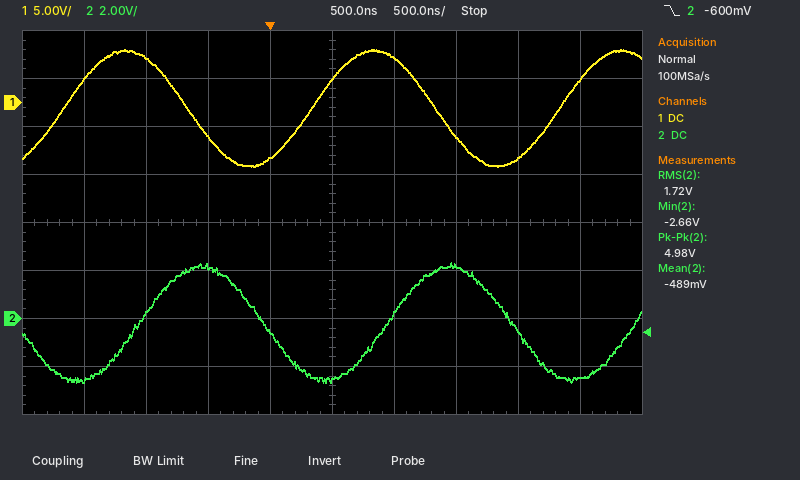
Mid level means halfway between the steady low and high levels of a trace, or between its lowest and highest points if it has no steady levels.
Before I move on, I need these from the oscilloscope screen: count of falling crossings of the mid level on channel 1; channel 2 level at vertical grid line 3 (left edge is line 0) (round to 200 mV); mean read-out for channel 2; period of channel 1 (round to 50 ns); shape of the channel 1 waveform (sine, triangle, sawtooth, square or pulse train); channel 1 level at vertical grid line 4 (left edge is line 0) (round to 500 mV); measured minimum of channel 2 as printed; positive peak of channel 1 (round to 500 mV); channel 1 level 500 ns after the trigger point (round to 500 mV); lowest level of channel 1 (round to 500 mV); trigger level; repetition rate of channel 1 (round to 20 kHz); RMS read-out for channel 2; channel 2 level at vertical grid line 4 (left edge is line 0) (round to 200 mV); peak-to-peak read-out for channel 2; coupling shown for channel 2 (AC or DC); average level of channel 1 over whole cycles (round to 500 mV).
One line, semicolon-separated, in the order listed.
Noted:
2; 2.2 V; -489 mV; 2.00 µs; sine; -6.0 V; -2.66 V; 5.5 V; 2.5 V; -6.5 V; -600 mV; 500 kHz; 1.72 V; -600 mV; 4.98 V; DC; -500 mV
